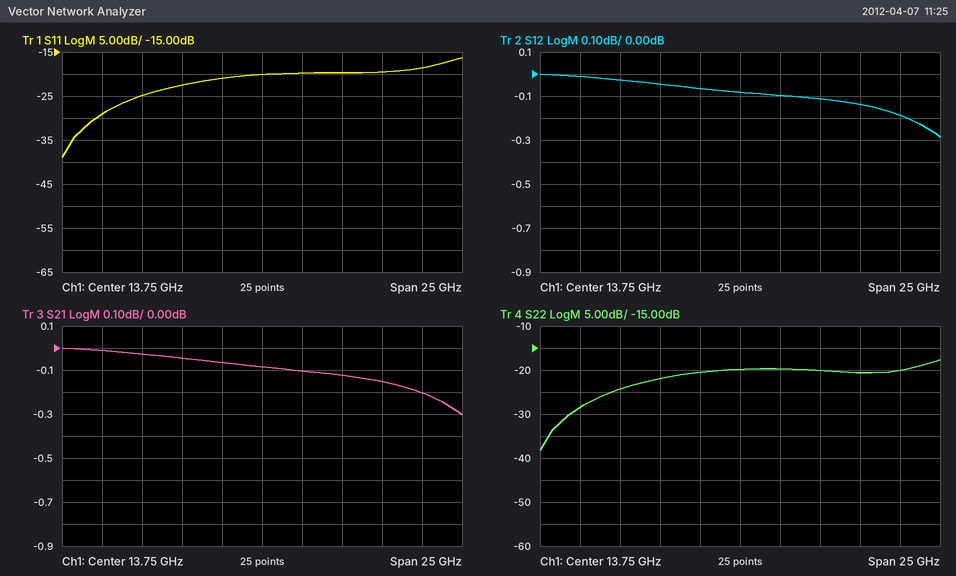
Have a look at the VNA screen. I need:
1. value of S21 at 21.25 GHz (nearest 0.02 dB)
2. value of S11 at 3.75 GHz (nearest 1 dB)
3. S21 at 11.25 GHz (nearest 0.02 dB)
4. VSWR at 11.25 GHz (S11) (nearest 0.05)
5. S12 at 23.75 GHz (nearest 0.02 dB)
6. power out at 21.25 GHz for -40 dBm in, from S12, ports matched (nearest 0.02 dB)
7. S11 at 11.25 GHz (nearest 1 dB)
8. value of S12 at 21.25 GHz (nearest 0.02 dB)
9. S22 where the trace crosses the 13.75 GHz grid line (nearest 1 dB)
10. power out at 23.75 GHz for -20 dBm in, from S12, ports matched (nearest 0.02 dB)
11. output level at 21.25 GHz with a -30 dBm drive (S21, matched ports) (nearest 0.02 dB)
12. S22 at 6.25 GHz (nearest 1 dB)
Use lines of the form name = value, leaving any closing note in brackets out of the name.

value of S21 at 21.25 GHz = -0.16 dB
value of S11 at 3.75 GHz = -29 dB
S21 at 11.25 GHz = -0.06 dB
VSWR at 11.25 GHz (S11) = 1.20
S12 at 23.75 GHz = -0.18 dB
power out at 21.25 GHz for -40 dBm in, from S12, ports matched = -40.14 dBm
S11 at 11.25 GHz = -21 dB
value of S12 at 21.25 GHz = -0.14 dB
S22 where the trace crosses the 13.75 GHz grid line = -20 dB
power out at 23.75 GHz for -20 dBm in, from S12, ports matched = -20.18 dBm
output level at 21.25 GHz with a -30 dBm drive (S21, matched ports) = -30.16 dBm
S22 at 6.25 GHz = -24 dB
